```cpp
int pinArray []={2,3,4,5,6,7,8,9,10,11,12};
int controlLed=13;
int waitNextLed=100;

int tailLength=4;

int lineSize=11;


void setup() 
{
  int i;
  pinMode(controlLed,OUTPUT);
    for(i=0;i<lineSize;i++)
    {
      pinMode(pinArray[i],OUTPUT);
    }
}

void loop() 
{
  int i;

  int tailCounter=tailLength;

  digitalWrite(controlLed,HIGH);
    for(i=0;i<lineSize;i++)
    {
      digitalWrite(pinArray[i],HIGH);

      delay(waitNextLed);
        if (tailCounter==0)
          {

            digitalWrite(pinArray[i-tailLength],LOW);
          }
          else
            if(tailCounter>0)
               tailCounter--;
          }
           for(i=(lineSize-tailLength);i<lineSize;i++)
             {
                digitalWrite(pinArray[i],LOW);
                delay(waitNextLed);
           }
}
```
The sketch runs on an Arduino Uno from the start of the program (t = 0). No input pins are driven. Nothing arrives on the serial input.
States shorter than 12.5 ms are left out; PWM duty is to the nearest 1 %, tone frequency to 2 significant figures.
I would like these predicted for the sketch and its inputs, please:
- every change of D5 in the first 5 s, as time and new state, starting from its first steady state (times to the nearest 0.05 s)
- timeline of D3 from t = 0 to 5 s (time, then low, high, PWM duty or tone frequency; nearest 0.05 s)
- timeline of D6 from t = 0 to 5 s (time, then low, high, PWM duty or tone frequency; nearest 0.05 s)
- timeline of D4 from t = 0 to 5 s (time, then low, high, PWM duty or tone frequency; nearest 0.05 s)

0 s low; 0.3 s high; 0.8 s low; 1.8 s high; 2.3 s low; 3.3 s high; 3.8 s low; 4.8 s high
0 s low; 0.1 s high; 0.6 s low; 1.6 s high; 2.1 s low; 3.1 s high; 3.6 s low; 4.6 s high
0 s low; 0.4 s high; 0.9 s low; 1.9 s high; 2.4 s low; 3.4 s high; 3.9 s low; 4.9 s high
0 s low; 0.2 s high; 0.7 s low; 1.7 s high; 2.2 s low; 3.2 s high; 3.7 s low; 4.7 s high
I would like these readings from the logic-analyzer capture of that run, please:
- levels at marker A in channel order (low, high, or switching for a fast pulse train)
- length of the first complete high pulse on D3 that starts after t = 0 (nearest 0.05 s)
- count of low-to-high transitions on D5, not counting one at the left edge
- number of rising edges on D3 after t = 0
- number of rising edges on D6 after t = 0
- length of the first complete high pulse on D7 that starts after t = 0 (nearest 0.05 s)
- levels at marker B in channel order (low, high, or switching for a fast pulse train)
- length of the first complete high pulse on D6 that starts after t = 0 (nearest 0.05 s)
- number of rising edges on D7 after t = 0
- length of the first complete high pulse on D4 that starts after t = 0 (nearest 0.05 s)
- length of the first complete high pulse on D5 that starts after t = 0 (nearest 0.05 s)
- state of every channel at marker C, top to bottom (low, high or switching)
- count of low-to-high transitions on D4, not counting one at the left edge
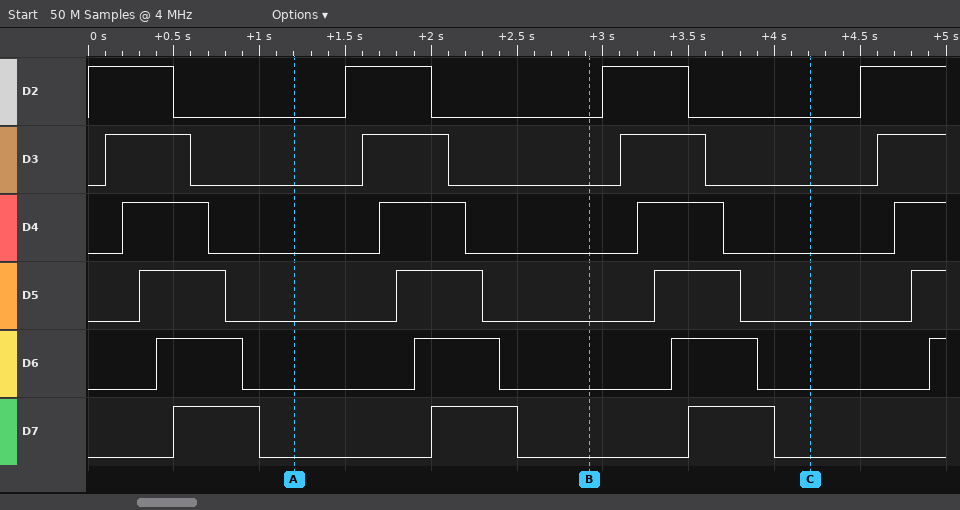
D2 low, D3 low, D4 low, D5 low, D6 low, D7 low
0.50 s
4
4
4
0.50 s
D2 low, D3 low, D4 low, D5 low, D6 low, D7 low
0.50 s
3
0.50 s
0.50 s
D2 low, D3 low, D4 low, D5 low, D6 low, D7 low
4
